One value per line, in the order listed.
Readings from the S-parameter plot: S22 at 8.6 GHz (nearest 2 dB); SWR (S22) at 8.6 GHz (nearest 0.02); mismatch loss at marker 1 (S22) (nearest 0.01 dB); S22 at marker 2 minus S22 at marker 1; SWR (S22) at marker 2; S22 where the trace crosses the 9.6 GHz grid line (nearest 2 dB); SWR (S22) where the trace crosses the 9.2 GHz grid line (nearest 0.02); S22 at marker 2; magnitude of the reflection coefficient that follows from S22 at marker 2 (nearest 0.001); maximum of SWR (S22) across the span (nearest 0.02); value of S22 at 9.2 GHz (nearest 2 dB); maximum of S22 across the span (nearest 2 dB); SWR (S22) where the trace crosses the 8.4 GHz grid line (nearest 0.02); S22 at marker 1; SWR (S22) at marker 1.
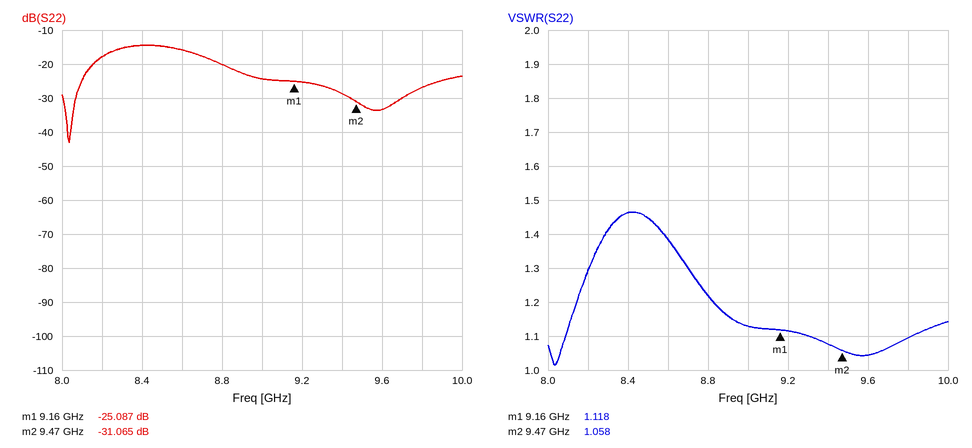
-16 dB
1.38
0.01 dB
-5.978 dB
1.058
-34 dB
1.12
-31.065 dB
0.028
1.46
-26 dB
-14 dB
1.46
-25.087 dB
1.118
